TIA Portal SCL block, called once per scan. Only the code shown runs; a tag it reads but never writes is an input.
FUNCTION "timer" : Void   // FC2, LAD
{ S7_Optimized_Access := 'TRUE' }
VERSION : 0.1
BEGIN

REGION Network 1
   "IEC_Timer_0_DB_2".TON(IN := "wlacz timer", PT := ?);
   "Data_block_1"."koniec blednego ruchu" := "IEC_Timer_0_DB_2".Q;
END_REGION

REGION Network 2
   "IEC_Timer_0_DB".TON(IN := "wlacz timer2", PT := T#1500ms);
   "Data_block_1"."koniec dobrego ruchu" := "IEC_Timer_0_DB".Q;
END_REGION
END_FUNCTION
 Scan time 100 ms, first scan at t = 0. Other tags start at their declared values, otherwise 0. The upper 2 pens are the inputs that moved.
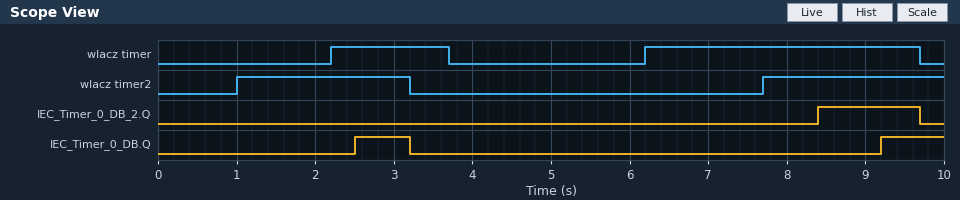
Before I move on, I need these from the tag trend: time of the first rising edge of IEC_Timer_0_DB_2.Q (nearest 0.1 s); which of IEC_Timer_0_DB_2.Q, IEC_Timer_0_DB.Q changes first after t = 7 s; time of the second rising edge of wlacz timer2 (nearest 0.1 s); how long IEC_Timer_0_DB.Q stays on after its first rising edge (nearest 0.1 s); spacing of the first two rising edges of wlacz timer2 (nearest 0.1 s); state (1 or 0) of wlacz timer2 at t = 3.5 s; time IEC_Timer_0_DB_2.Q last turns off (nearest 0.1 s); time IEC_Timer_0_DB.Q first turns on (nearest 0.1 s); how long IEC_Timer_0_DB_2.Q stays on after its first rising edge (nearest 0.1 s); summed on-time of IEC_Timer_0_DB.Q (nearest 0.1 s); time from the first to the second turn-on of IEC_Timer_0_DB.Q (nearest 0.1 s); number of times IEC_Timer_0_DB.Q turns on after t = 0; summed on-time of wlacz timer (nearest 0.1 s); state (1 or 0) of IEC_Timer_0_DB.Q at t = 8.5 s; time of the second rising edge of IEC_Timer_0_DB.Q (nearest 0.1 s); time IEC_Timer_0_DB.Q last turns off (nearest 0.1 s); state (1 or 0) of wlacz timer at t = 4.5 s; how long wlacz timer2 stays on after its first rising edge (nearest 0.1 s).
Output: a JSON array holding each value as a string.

["8.4 s", "IEC_Timer_0_DB_2.Q", "7.7 s", "0.7 s", "6.7 s", "0", "9.7 s", "2.5 s", "1.3 s", "1.5 s", "6.7 s", "2", "5.0 s", "0", "9.2 s", "3.2 s", "0", "2.2 s"]
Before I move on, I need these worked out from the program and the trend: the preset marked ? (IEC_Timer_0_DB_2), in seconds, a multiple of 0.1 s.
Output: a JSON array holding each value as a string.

["2.2 s"]
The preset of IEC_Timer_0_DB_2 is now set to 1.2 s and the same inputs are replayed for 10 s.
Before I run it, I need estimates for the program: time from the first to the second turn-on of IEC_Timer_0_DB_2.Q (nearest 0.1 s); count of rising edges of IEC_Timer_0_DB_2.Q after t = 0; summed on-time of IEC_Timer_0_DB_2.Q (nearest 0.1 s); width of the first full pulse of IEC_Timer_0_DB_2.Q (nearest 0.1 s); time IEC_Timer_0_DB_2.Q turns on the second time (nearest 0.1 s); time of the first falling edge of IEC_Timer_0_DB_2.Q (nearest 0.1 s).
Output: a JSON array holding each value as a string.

["4.0 s", "2", "2.6 s", "0.3 s", "7.4 s", "3.7 s"]
